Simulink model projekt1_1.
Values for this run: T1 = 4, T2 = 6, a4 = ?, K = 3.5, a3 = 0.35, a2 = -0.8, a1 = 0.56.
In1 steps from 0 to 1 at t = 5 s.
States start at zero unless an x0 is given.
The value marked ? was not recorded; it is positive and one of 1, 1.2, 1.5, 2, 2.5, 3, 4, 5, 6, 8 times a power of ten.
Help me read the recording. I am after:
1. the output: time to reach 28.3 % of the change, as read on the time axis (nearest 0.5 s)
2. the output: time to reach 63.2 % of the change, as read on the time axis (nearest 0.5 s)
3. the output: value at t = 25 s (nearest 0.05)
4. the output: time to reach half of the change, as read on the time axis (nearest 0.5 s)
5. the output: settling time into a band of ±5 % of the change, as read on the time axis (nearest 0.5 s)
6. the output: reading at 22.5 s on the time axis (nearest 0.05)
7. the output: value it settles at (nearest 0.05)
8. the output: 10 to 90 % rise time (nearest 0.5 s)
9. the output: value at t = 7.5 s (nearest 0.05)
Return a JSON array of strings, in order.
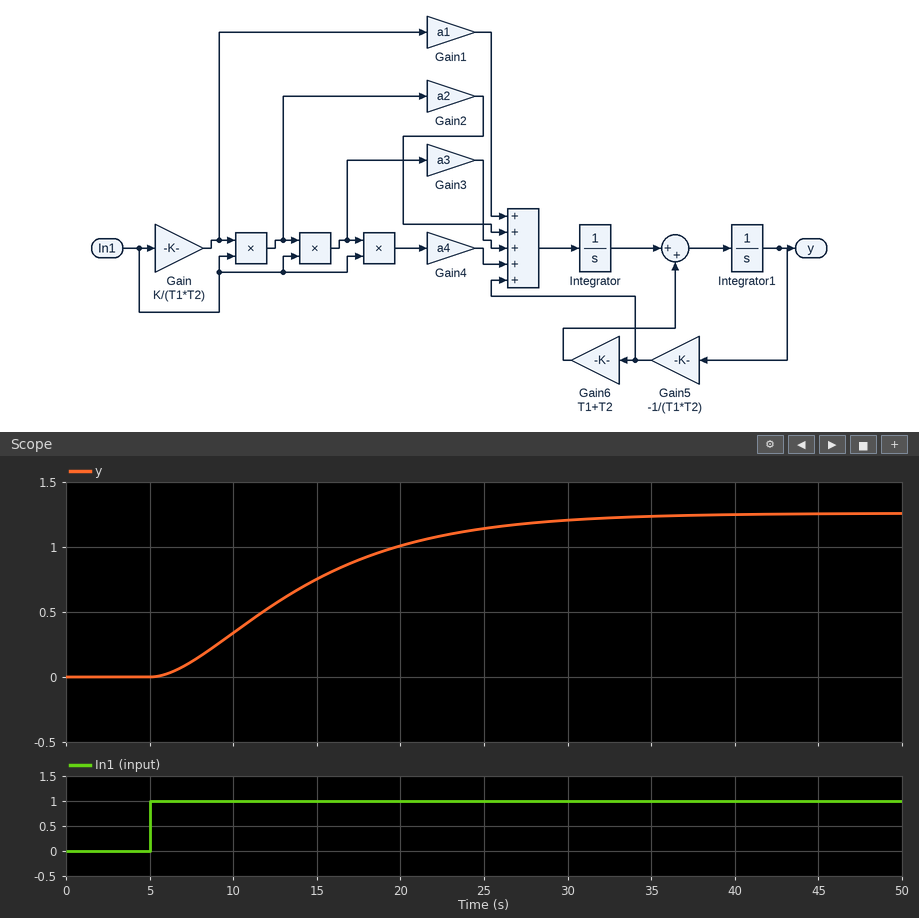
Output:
["10.0 s", "15.5 s", "1.15", "13.5 s", "29.0 s", "1.10", "1.25", "17.0 s", "0.10"]
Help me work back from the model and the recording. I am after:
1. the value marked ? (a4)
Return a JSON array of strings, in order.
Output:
["0.25"]
